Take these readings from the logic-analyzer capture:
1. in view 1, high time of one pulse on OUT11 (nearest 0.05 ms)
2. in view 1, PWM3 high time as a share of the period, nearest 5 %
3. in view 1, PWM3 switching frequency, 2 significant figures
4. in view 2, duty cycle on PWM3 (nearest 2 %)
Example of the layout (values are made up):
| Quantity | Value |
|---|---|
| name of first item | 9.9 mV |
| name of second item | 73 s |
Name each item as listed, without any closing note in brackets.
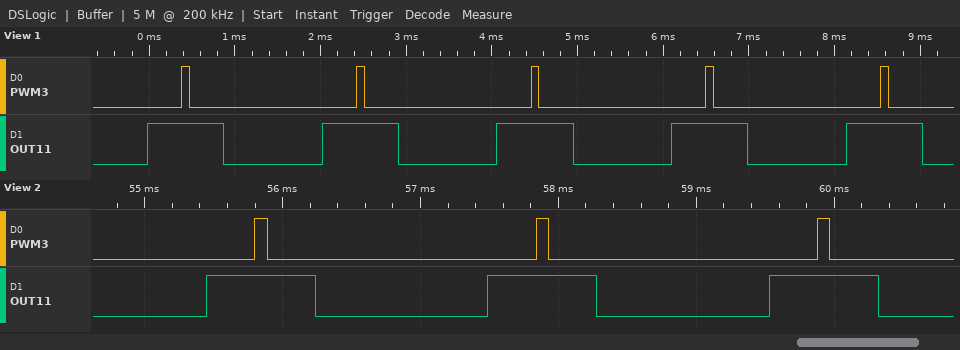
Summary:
| Quantity | Value |
|---|---|
| in view 1, high time of one pulse on OUT11 | 0.90 ms |
| in view 1, PWM3 high time as a share of the period, nearest 5 % | 5 % |
| in view 1, PWM3 switching frequency, 2 significant figures | 490 Hz |
| in view 2, duty cycle on PWM3 | 4 % |
